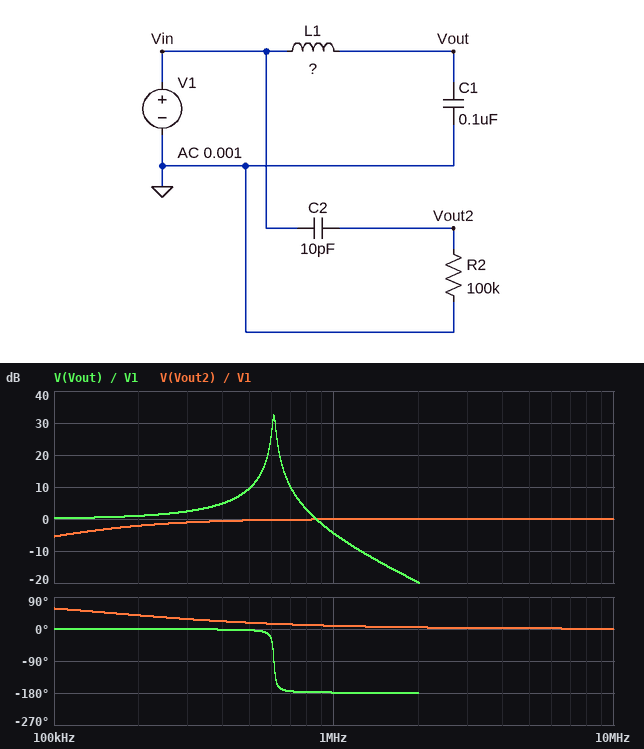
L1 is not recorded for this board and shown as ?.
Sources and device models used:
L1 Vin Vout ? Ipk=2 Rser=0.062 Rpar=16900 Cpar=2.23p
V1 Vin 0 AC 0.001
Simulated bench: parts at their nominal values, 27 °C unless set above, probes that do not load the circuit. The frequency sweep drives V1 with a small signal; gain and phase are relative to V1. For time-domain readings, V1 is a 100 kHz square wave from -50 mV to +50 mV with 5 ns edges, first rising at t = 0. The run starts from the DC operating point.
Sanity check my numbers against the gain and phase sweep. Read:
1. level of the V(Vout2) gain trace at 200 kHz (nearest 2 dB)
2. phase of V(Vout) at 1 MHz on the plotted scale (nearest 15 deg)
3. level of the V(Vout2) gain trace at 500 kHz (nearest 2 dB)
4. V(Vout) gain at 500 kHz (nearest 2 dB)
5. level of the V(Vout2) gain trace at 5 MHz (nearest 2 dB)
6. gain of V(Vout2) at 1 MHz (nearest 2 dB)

-2 dB
-180 deg
0 dB
10 dB
0 dB
0 dB
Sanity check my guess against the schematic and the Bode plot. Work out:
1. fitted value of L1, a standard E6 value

680 nH
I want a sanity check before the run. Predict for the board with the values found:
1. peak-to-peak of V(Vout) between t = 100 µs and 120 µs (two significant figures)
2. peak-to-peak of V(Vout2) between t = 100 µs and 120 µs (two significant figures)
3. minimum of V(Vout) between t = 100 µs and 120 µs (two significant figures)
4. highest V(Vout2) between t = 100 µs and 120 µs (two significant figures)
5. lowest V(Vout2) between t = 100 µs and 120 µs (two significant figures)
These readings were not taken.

210 mV
200 mV
-100 mV
99 mV
-99 mV
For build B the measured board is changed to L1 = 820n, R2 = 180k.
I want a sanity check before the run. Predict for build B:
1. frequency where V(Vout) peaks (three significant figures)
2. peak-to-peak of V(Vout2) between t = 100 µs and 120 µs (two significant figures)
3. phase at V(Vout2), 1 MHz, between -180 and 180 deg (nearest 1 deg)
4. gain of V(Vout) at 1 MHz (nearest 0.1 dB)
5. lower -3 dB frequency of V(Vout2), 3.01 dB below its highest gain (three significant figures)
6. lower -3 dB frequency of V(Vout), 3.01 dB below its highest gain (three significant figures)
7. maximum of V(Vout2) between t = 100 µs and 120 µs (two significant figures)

556 kHz
190 mV
5 deg
-7.0 dB
88.4 kHz
550 kHz
94 mV
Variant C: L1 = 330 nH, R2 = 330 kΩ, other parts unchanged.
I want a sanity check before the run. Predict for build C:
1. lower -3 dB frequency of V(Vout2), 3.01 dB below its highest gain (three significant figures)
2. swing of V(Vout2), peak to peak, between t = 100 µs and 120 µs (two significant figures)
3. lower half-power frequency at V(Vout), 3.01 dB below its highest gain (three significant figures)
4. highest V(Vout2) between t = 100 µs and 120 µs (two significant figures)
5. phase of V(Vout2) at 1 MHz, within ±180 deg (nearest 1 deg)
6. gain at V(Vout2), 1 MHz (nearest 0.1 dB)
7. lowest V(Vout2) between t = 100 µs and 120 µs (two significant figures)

48.2 kHz
160 mV
861 kHz
82 mV
3 deg
0 dB
-82 mV
